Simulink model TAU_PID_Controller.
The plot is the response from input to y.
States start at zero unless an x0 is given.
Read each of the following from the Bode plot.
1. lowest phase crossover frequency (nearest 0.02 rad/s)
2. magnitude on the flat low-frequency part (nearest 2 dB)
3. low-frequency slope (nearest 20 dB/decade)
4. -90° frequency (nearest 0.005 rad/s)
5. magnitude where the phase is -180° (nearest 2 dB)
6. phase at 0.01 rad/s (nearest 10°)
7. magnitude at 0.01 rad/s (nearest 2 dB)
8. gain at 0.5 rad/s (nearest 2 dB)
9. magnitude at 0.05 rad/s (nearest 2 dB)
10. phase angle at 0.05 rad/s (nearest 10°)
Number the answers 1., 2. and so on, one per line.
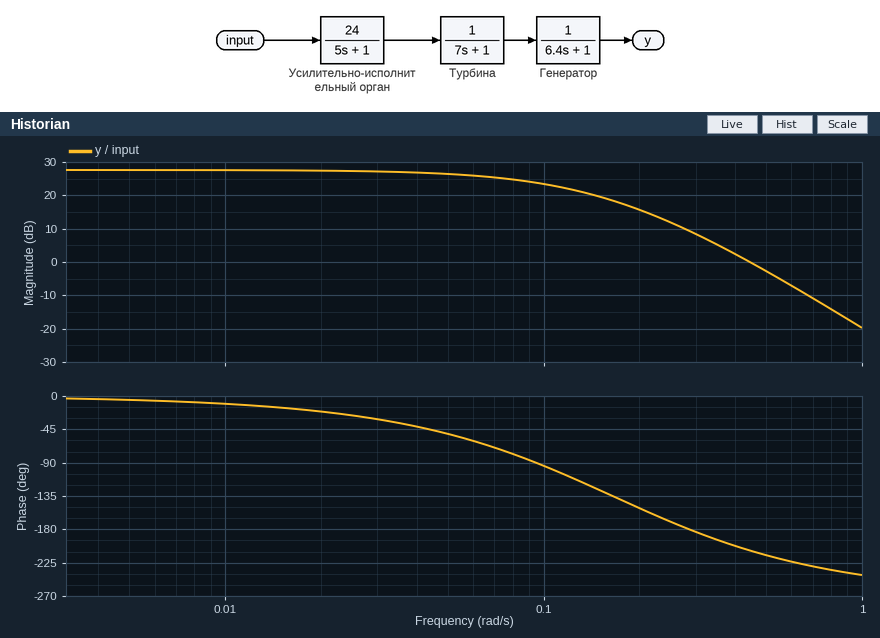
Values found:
1. 0.28 rad/s
2. 28 dB
3. 0 dB/decade
4. 0.095 rad/s
5. 10 dB
6. -10°
7. 28 dB
8. -2 dB
9. 26 dB
10. -50°
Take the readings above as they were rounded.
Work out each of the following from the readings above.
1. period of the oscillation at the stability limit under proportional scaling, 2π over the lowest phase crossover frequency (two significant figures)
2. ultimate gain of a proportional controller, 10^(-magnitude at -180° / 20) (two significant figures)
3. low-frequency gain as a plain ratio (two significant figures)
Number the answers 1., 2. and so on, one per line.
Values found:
1. 22 s
2. 0.32
3. 25
